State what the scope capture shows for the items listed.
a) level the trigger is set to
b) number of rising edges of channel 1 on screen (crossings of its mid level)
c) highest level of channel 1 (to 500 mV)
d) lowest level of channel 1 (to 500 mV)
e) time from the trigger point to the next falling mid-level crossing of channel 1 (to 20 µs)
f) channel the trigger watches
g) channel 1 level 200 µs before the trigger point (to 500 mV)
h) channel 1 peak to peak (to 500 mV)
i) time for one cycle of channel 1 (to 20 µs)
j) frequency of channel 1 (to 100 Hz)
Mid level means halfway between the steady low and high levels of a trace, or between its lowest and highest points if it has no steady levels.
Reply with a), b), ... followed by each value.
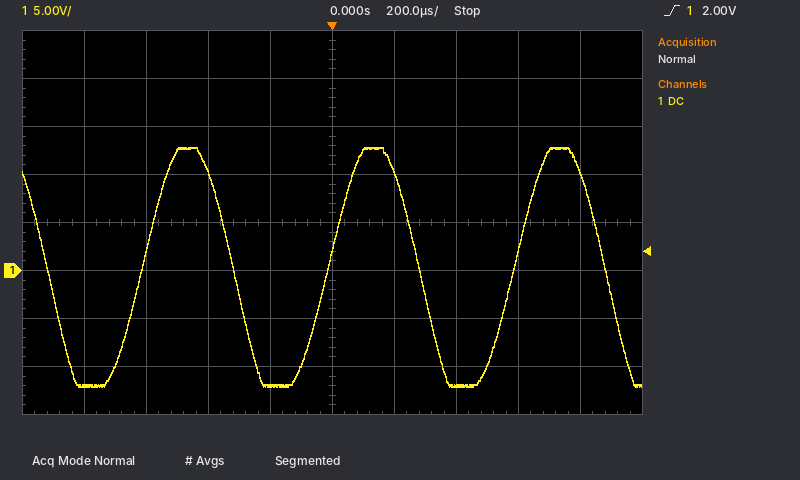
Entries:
a) 2.00 V
b) 3
c) 13.0 V
d) -12.0 V
e) 280 µs
f) channel 1
g) -12.0 V
h) 25.0 V
i) 600 µs
j) 1.7 kHz
